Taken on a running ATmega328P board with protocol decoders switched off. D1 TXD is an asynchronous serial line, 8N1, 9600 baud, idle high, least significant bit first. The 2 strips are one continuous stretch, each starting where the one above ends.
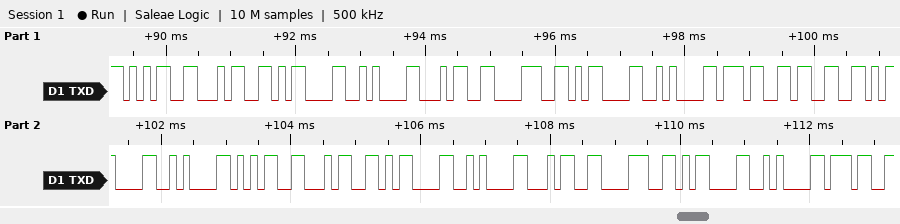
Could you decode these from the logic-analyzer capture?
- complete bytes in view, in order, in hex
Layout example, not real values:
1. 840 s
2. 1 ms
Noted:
1. 0x35 0x34 0x0D 0x0A 0x34 0x38 0x0D 0x0A 0x37 0x33 0x0D 0x0A 0x35 0x34 0x0D 0x0A 0x34 0x38 0x0D 0x0A 0x37
